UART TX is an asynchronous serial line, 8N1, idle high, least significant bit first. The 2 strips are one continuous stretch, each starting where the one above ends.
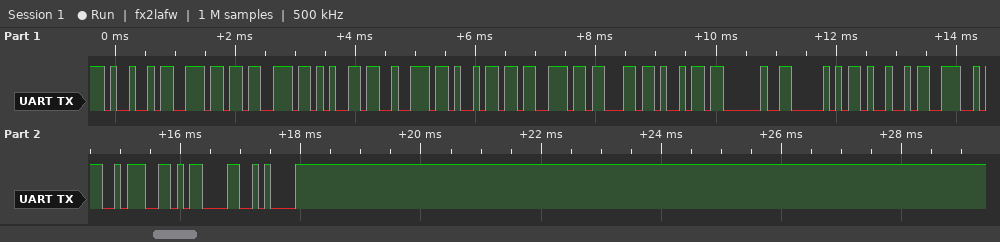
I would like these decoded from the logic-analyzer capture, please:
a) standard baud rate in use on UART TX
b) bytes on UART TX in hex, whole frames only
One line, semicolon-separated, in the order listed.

9600 baud; 49 6E 73 65 72 69 73 63 69 20 50 49 4E 3A 0D 0A
